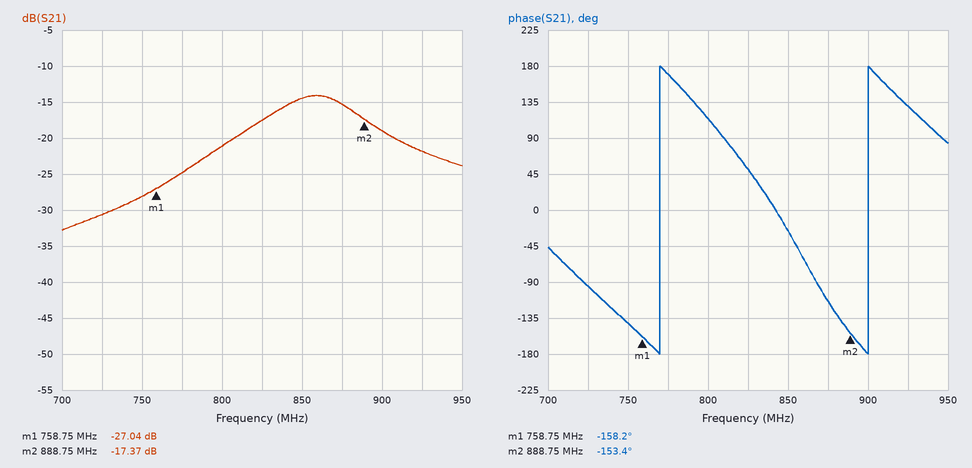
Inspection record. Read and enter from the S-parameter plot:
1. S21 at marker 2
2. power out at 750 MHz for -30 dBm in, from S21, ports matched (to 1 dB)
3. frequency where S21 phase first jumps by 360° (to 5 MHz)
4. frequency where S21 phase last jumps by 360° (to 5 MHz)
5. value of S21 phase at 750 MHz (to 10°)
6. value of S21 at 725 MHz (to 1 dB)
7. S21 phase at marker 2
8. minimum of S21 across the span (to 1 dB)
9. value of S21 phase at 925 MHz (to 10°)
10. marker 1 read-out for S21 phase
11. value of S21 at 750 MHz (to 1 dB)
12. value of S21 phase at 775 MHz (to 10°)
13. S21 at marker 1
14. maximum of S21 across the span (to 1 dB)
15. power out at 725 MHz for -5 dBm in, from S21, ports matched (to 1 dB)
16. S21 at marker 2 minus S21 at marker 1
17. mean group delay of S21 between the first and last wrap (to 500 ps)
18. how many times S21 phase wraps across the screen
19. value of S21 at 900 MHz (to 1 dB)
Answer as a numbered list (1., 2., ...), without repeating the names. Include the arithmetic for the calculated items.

1. -17.37 dB
2. -30 dBm + (-28 dB) = -58 dBm
3. 770 MHz
4. 900 MHz
5. -140°
6. -31 dB
7. -153.4°
8. -33 dB
9. 130°
10. -158.2°
11. -28 dB
12. 170°
13. -27.04 dB
14. -14 dB
15. -5 dBm + (-31 dB) = -36 dBm
16. -17.37 − (-27.04) = 9.67 dB
17. 1 cycle / (900 MHz − 770 MHz) ≈ 7.69 ns, so 7.5 ns to the nearest 500 ps
18. 2
19. -19 dB
